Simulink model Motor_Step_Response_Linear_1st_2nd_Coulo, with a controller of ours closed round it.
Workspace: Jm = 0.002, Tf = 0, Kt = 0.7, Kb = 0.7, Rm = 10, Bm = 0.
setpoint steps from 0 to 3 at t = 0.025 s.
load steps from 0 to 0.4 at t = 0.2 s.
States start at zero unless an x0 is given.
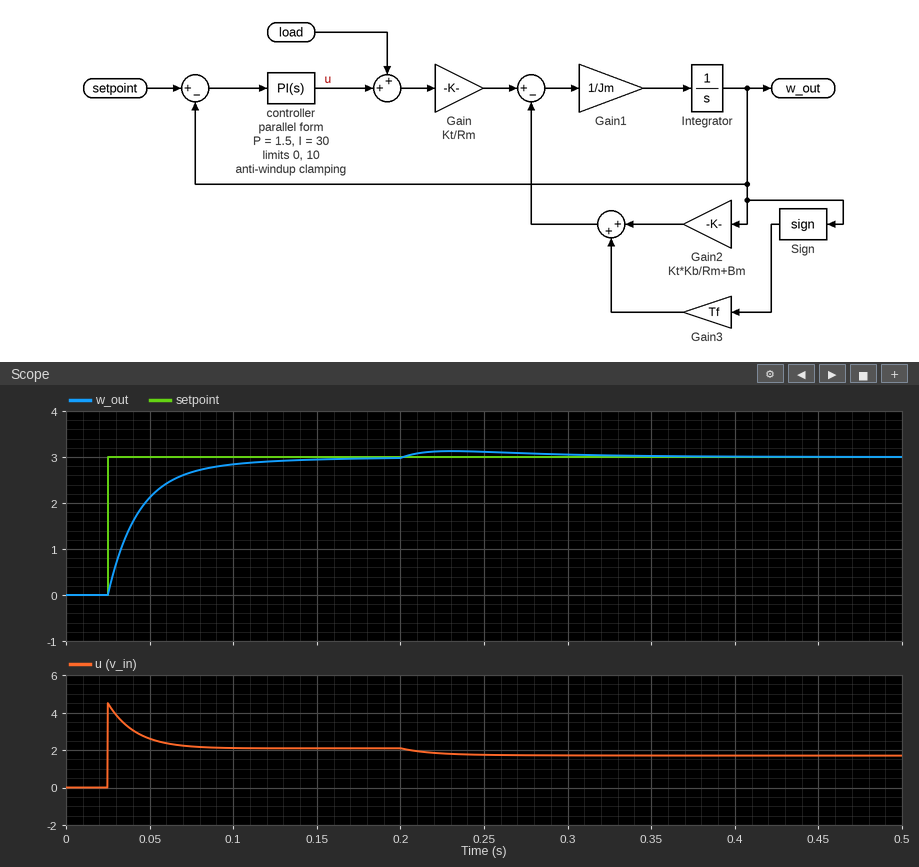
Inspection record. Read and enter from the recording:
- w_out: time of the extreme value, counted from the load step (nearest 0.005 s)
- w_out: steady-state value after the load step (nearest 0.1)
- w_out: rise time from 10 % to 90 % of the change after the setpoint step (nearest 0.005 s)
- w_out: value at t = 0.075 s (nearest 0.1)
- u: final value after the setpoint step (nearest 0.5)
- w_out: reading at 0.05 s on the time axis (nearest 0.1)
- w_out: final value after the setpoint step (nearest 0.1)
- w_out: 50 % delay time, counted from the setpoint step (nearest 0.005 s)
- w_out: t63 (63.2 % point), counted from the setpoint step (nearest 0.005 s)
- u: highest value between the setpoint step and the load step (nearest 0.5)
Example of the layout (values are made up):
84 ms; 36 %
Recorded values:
0.030 s; 3.0; 0.050 s; 2.7; 2.0; 2.1; 3.0; 0.015 s; 0.020 s; 4.5
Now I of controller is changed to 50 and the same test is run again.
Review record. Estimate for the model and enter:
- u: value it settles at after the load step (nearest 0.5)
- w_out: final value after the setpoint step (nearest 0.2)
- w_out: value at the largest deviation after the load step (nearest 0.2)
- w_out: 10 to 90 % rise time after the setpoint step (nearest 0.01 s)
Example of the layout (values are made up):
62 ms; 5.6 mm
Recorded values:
1.5; 3.0; 3.2; 0.03 s
